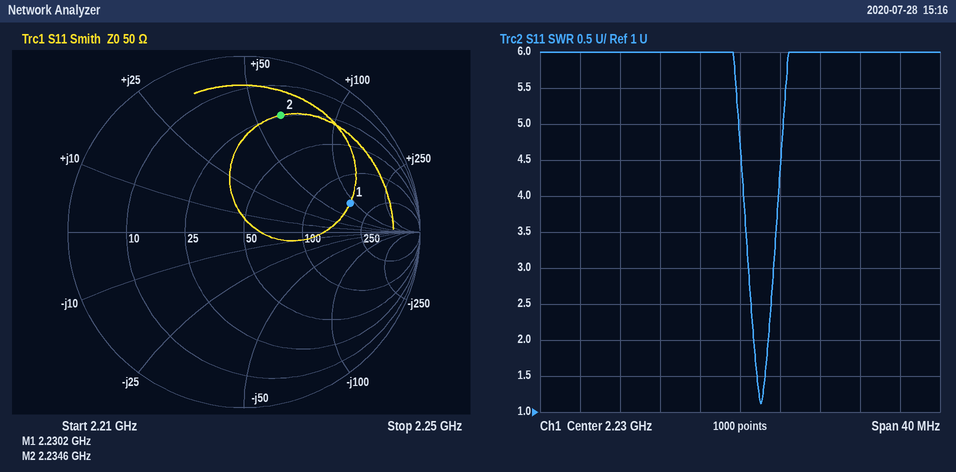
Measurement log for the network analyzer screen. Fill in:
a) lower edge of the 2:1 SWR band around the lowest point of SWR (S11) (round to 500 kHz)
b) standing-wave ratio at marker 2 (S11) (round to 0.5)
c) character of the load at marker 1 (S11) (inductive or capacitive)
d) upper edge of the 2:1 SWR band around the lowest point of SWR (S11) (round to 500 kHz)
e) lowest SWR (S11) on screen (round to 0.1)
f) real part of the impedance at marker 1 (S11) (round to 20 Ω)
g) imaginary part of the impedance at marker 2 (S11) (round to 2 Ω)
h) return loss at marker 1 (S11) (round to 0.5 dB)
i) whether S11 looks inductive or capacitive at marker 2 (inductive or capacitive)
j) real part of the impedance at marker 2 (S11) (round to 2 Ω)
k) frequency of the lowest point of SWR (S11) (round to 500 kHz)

2.2315 GHz
5.5
inductive
2.2330 GHz
1.1
160 Ω
+62 Ω
4.0 dB
inductive
24 Ω
2.2320 GHz
